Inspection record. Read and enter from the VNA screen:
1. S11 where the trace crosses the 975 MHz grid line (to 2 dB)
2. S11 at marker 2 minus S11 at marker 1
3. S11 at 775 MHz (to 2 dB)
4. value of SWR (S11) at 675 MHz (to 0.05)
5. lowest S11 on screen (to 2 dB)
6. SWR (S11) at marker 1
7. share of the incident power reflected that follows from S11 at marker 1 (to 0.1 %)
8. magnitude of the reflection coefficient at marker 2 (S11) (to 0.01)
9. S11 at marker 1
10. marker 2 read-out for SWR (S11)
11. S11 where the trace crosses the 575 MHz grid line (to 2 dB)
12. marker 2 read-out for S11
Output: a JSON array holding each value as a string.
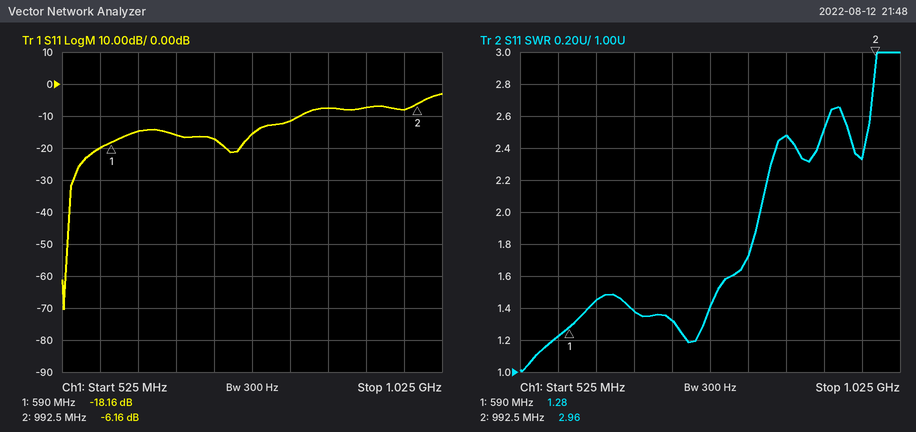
["-8 dB", "12.00 dB", "-16 dB", "1.40", "-70 dB", "1.28", "1.5 %", "0.49", "-18.16 dB", "2.96", "-20 dB", "-6.16 dB"]
